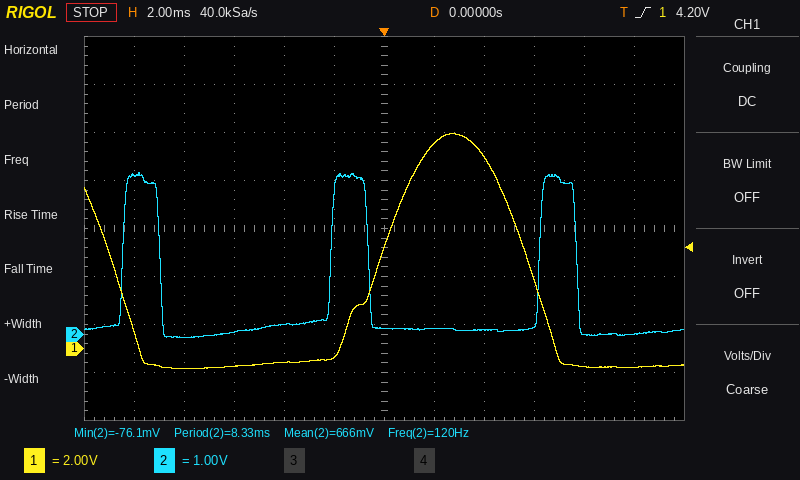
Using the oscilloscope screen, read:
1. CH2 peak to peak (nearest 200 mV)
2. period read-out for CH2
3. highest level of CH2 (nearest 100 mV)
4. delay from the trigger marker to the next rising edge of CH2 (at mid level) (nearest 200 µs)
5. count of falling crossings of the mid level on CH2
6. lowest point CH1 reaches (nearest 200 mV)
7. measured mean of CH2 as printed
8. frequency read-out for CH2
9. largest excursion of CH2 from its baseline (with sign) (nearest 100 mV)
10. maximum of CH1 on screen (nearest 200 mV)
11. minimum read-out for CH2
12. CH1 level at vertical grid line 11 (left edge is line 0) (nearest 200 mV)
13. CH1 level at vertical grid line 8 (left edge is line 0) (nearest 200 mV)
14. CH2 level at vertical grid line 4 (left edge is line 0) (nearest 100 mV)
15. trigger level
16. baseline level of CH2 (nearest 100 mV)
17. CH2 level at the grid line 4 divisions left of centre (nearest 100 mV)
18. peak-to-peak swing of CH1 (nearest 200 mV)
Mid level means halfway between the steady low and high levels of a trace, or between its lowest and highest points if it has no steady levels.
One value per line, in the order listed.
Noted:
3.4 V
8.33 ms
3.4 V
6.2 ms
3
-800 mV
666 mV
120 Hz
+3.3 V
9.0 V
-76.1 mV
-800 mV
8.0 V
200 mV
4.20 V
100 mV
-100 mV
9.8 V
